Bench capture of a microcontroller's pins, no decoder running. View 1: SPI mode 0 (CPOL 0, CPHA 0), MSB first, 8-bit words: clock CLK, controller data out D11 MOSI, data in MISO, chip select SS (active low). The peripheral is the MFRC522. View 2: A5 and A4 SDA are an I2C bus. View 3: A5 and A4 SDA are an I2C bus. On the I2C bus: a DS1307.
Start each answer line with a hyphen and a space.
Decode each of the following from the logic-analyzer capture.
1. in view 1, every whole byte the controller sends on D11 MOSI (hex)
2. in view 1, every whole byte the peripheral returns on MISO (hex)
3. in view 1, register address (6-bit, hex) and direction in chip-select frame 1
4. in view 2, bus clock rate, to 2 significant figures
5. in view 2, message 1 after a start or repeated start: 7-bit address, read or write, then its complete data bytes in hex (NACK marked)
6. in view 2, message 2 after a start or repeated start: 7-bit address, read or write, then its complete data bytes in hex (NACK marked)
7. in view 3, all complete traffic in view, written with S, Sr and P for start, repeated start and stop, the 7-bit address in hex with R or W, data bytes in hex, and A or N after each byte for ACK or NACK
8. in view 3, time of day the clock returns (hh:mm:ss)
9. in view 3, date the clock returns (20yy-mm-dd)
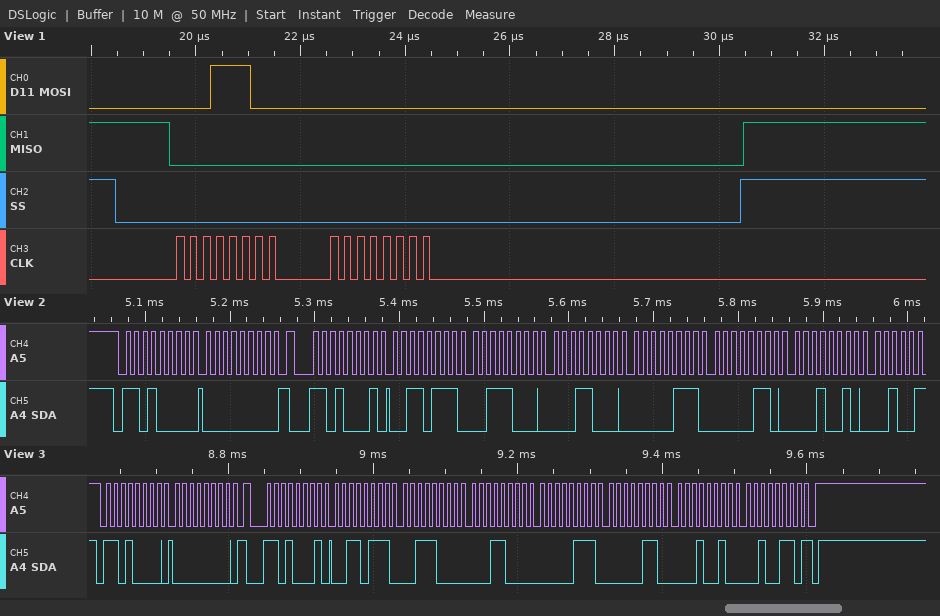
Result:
- 1C 00
- 00 00
- 0x0E write
- 100 kHz
- 0x68 write: 00
- 0x68 read: 37 38 18 07 06 12
- S 68W A 00 A Sr 68R A 37 A 38 A 18 A 07 A 06 A 12 A 26 N P
- 18:38:37
- 2026-12-06
